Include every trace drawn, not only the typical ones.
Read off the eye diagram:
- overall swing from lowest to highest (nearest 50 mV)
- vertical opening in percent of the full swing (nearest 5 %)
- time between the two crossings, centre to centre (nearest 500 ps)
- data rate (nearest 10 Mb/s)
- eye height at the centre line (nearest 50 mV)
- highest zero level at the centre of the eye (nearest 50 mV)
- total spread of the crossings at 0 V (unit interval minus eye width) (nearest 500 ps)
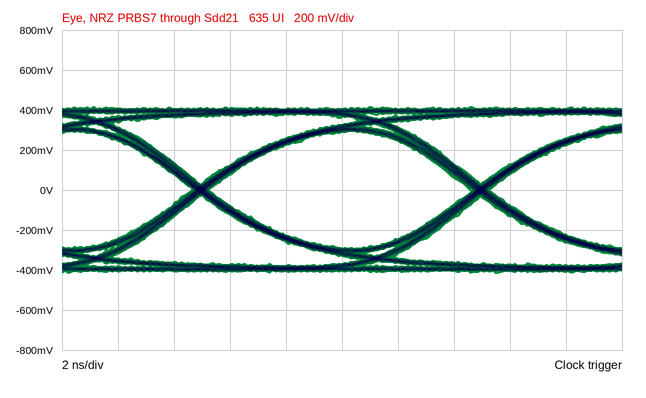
850 mV
70 %
10.0 ns
100 Mb/s
600 mV
-300 mV
500 ps
